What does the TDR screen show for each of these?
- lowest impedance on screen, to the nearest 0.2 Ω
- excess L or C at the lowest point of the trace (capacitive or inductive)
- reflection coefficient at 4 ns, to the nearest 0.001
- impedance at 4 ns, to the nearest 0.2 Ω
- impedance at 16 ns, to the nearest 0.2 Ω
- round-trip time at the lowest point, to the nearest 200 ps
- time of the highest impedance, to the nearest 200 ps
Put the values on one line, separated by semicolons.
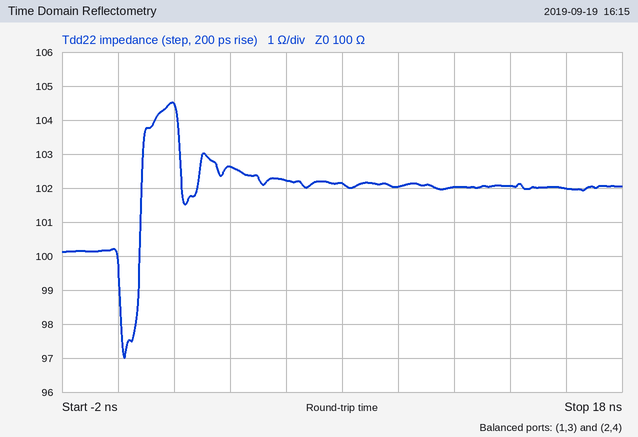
97.0 Ω; capacitive; +0.013; 102.6 Ω; 102.0 Ω; 200 ps; 2.0 ns
